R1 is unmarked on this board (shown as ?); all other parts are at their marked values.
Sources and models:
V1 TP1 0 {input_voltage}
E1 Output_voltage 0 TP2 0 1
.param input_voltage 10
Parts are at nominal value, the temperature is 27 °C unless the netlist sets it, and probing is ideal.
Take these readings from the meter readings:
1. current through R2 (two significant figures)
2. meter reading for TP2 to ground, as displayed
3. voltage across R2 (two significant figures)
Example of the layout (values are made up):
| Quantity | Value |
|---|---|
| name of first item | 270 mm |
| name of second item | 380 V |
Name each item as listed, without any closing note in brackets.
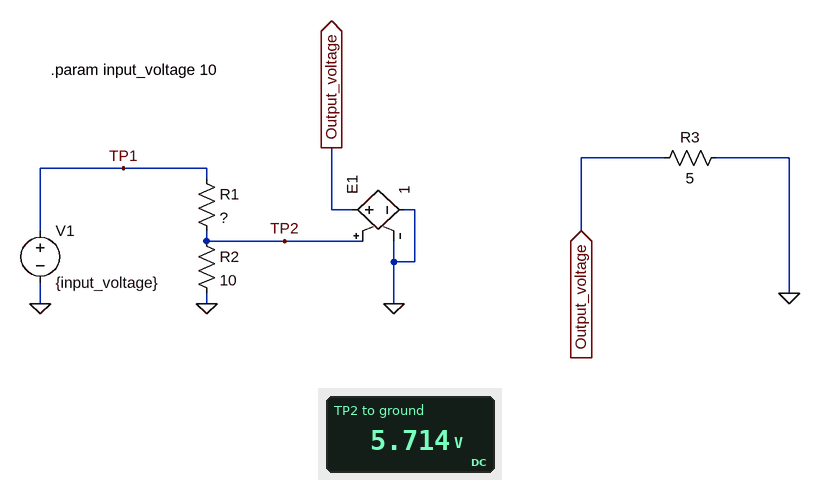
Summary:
| Quantity | Value |
|---|---|
| current through R2 | 570 mA |
| meter reading for TP2 to ground, as displayed | 5.714 V |
| voltage across R2 | 5.7 V |
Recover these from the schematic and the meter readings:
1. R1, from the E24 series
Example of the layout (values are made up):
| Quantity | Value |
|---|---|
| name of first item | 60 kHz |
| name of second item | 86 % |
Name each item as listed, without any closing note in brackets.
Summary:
| Quantity | Value |
|---|---|
| R1, from the E24 series | 7.5 Ω |
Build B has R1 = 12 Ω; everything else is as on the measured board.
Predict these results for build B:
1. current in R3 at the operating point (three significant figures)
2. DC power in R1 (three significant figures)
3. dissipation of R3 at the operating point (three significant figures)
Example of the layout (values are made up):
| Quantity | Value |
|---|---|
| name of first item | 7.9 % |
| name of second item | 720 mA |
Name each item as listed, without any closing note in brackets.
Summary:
| Quantity | Value |
|---|---|
| current in R3 at the operating point | 909 mA |
| DC power in R1 | 2.48 W |
| dissipation of R3 at the operating point | 4.13 W |
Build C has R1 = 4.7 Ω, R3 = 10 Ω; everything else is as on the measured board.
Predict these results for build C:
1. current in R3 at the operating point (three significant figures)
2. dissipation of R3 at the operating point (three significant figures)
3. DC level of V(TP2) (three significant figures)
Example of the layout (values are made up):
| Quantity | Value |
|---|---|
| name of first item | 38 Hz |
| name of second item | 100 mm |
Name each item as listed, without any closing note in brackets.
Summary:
| Quantity | Value |
|---|---|
| current in R3 at the operating point | 680 mA |
| dissipation of R3 at the operating point | 4.63 W |
| DC level of V(TP2) | 6.80 V |
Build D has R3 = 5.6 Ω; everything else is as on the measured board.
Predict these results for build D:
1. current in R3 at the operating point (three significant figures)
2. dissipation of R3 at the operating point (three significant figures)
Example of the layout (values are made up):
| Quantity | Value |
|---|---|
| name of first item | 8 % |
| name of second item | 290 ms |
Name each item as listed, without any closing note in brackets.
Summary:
| Quantity | Value |
|---|---|
| current in R3 at the operating point | 1.02 A |
| dissipation of R3 at the operating point | 5.83 W |
